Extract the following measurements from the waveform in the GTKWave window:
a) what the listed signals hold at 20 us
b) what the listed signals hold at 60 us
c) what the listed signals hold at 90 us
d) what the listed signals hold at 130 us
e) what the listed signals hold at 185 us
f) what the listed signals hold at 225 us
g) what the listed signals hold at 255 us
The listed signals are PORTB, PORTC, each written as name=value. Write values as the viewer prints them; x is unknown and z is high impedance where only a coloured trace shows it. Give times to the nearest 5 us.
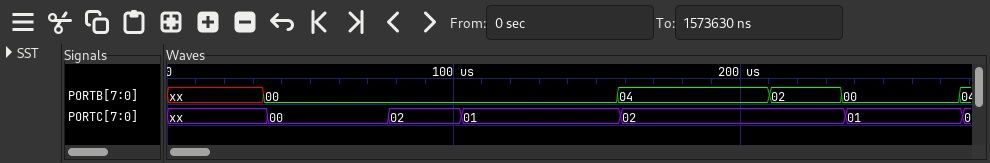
PORTB=xx, PORTC=xx
PORTB=00, PORTC=00
PORTB=00, PORTC=02
PORTB=00, PORTC=01
PORTB=04, PORTC=02
PORTB=02, PORTC=02
PORTB=00, PORTC=01
